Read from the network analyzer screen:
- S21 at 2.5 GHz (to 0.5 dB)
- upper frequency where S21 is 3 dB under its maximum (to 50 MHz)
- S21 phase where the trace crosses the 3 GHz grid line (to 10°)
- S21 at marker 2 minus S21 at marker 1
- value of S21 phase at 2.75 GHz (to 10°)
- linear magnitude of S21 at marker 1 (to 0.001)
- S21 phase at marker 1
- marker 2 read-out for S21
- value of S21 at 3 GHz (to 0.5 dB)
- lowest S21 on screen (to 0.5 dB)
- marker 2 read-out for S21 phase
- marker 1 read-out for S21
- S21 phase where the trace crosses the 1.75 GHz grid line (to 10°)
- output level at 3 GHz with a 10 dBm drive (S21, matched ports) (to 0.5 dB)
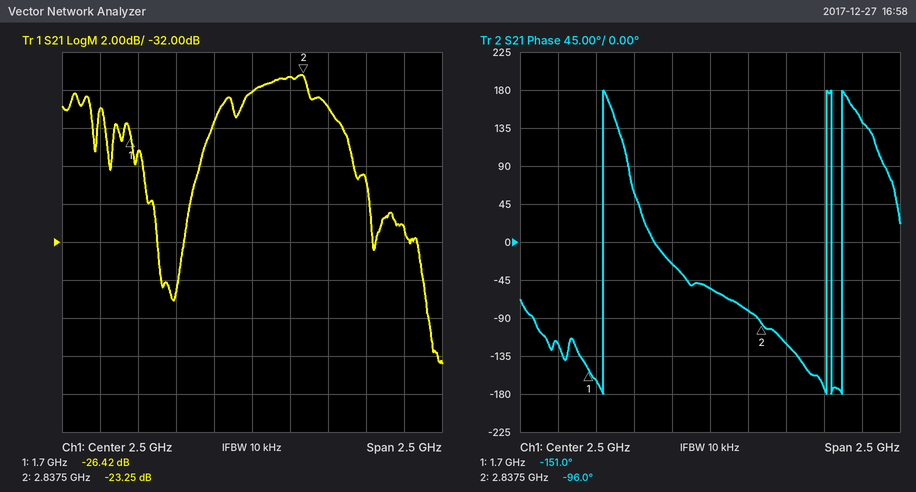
-24.0 dB
3.10 GHz
-120°
3.17 dB
-80°
0.048
-151.0°
-23.25 dB
-25.0 dB
-38.5 dB
-96.0°
-26.42 dB
-160°
-15.0 dBm
